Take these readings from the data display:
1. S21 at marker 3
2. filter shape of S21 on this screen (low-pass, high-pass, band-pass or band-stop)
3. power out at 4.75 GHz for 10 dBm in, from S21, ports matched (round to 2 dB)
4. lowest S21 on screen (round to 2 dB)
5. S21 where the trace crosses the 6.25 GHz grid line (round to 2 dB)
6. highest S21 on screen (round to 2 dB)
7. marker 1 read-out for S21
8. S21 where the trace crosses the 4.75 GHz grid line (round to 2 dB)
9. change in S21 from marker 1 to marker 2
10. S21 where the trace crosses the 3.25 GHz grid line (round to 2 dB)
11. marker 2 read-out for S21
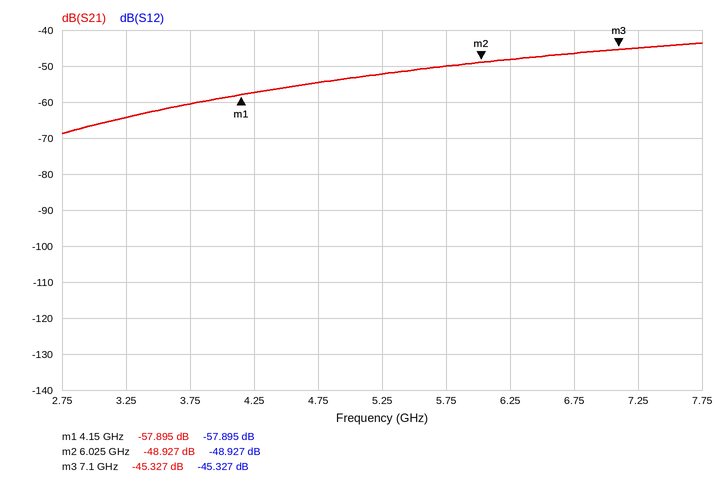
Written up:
-45.327 dB
high-pass
-44 dBm
-68 dB
-48 dB
-44 dB
-57.895 dB
-54 dB
8.968 dB
-64 dB
-48.927 dB
